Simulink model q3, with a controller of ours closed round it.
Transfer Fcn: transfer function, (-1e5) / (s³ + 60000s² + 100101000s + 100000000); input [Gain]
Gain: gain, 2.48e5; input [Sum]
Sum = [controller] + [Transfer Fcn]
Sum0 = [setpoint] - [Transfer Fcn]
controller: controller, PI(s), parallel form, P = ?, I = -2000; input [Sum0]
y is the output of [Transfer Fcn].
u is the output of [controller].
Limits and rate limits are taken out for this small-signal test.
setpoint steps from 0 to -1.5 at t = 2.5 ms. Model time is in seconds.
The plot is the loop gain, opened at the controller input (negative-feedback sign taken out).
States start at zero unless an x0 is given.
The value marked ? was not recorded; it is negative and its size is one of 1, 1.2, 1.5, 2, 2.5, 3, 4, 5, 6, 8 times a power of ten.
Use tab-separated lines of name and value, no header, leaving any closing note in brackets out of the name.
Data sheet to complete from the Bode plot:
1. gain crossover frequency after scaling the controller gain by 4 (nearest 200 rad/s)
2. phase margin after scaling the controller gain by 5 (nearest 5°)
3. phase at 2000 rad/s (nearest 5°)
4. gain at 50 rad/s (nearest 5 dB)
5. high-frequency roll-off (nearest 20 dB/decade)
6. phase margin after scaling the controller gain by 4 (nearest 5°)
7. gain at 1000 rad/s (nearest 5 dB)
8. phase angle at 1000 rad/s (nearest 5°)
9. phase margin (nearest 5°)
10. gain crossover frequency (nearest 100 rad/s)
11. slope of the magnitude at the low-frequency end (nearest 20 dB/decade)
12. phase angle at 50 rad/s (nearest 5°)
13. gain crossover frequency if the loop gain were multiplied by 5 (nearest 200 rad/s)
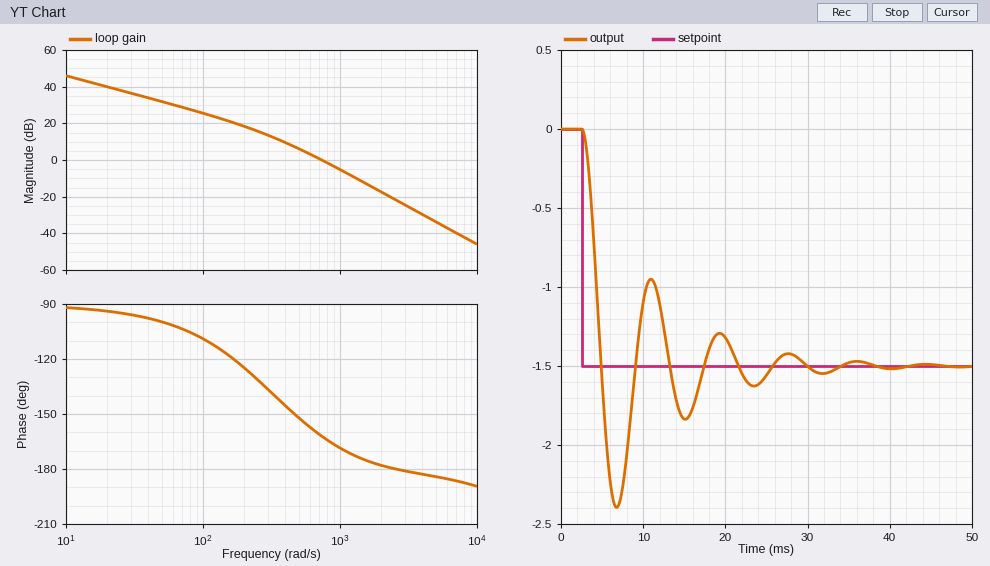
gain crossover frequency after scaling the controller gain by 4	1400 rad/s
phase margin after scaling the controller gain by 5	5°
phase at 2000 rad/s	-180°
gain at 50 rad/s	30 dB
high-frequency roll-off	-40 dB/decade
phase margin after scaling the controller gain by 4	5°
gain at 1000 rad/s	-5 dB
phase angle at 1000 rad/s	-170°
phase margin	20°
gain crossover frequency	700 rad/s
slope of the magnitude at the low-frequency end	-20 dB/decade
phase angle at 50 rad/s	-100°
gain crossover frequency if the loop gain were multiplied by 5	1600 rad/s
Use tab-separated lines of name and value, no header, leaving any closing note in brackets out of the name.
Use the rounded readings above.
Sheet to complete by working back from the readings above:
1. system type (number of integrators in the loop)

system type	1
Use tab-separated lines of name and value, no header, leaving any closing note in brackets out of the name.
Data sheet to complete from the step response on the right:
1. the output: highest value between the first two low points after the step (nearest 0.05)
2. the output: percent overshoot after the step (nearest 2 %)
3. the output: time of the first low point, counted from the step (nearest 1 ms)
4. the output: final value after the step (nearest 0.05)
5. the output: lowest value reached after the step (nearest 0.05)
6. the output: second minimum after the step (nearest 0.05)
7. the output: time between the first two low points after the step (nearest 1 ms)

the output: highest value between the first two low points after the step	-0.95
the output: percent overshoot after the step	60 %
the output: time of the first low point, counted from the step	4 ms
the output: final value after the step	-1.50
the output: lowest value reached after the step	-2.40
the output: second minimum after the step	-1.85
the output: time between the first two low points after the step	8 ms
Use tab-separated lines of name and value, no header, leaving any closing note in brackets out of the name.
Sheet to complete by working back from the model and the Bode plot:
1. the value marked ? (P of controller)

the value marked ?	-1.2
